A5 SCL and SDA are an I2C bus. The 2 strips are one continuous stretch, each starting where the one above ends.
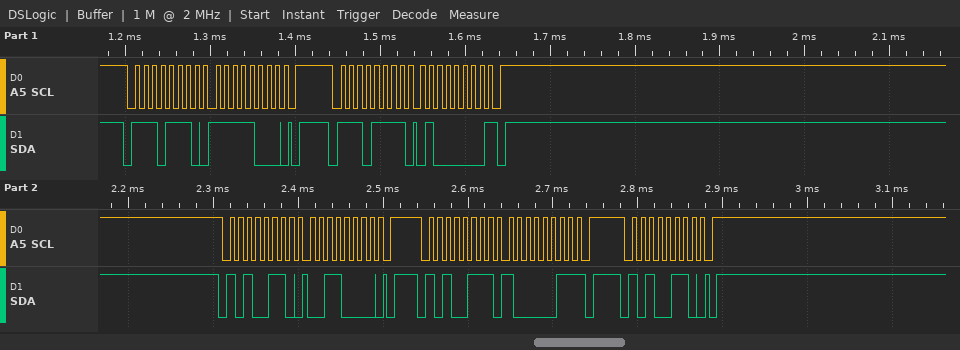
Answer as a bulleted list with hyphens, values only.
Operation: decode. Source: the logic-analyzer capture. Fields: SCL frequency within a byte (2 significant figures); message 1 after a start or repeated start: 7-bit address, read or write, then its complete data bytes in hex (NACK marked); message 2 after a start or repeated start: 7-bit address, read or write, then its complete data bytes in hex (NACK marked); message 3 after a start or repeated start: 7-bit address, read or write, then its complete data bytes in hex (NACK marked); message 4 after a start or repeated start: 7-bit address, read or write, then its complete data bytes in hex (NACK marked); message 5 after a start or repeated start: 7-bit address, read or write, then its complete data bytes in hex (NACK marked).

- 100 kHz
- 0x77 write: F8
- 0x77 read: 40 NACK
- 0x53 write: 30
- 0x53 read: 83 NACK
- 0x53 write
